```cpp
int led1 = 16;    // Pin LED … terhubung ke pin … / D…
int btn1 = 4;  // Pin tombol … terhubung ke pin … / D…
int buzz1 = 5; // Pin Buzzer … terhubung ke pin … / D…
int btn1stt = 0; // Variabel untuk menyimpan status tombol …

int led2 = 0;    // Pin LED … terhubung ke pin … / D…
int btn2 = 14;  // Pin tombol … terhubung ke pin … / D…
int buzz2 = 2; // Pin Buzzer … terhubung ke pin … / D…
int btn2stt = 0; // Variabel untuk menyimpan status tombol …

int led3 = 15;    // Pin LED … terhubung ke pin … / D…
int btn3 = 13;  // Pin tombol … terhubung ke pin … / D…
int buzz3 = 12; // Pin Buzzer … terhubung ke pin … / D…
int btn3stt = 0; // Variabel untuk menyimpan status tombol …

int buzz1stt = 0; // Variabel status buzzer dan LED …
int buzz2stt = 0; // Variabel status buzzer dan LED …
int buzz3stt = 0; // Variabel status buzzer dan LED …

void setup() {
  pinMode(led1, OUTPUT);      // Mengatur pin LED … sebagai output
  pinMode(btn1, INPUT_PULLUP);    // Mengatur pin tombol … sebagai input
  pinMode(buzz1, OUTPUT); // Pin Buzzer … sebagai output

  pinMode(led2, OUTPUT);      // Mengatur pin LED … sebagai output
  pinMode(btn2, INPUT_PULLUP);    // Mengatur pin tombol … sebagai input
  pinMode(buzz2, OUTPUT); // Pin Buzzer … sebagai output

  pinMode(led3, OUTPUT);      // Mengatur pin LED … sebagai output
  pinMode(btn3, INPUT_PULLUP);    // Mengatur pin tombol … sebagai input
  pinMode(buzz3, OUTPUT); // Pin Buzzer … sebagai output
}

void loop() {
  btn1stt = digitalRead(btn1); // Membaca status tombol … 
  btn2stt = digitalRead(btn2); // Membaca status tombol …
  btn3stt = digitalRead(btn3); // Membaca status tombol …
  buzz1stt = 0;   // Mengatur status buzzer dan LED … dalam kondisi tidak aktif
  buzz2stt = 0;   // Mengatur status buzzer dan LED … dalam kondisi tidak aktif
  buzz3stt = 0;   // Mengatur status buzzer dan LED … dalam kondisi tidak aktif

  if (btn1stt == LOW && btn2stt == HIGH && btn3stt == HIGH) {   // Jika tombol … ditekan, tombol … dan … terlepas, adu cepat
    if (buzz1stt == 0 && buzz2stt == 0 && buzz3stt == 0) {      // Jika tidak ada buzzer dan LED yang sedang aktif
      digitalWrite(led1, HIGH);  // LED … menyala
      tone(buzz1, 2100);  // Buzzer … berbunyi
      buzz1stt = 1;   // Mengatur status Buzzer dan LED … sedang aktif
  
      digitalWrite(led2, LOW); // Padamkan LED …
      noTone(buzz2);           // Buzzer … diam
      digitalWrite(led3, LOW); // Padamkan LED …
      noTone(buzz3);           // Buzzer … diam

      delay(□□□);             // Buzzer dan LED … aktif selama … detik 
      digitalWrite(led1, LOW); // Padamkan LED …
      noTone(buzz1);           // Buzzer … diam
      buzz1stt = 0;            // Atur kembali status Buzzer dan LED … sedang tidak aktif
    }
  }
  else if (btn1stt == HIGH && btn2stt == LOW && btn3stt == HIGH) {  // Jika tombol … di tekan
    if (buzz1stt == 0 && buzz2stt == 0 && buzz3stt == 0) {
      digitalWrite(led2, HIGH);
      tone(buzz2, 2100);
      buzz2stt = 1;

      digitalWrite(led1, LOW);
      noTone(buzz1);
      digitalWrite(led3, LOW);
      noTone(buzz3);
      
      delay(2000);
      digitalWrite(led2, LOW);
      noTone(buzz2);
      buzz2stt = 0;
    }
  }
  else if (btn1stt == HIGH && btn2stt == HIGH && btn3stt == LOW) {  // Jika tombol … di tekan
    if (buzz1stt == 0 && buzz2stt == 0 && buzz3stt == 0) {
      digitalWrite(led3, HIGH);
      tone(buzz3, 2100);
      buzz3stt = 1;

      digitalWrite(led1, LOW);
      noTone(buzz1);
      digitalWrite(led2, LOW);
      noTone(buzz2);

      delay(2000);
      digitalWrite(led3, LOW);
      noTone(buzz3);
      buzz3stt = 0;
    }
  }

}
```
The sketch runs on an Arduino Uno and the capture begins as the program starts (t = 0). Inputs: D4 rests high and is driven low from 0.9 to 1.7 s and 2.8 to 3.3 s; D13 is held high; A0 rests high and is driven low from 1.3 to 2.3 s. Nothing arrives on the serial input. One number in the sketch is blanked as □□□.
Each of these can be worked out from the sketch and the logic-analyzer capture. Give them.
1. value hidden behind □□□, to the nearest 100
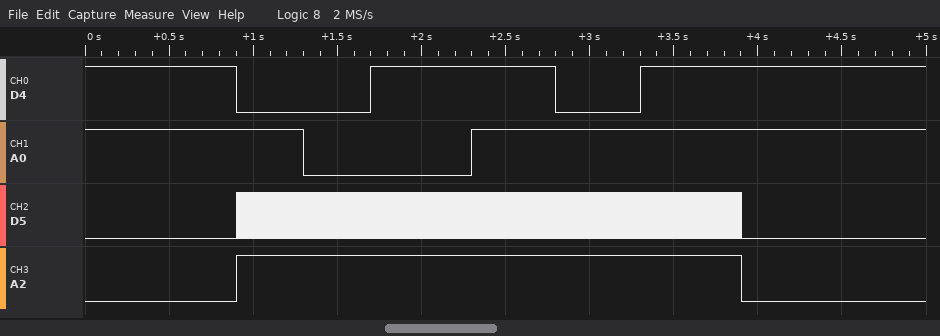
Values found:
3000
